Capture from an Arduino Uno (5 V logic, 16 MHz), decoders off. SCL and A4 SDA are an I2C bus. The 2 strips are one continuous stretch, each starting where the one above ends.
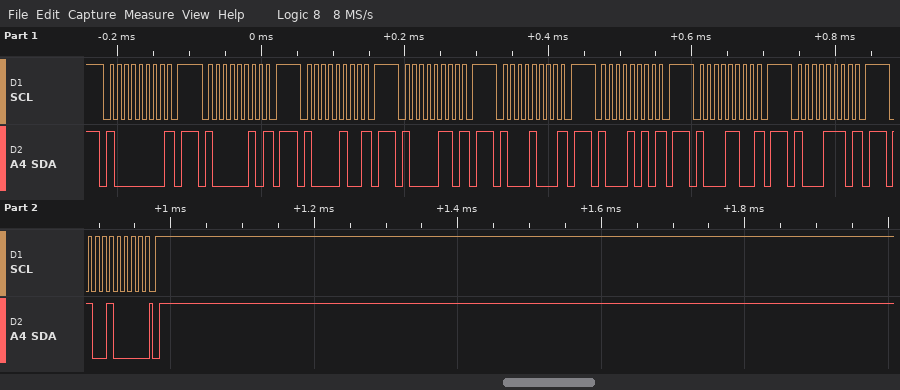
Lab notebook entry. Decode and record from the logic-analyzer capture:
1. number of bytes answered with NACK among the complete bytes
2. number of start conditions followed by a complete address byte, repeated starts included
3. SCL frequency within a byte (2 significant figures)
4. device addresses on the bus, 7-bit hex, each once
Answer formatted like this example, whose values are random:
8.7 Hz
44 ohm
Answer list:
8
9
100 kHz
0x40 0x41 0x42 0x43 0x44 0x45 0x46 0x47 0x48
